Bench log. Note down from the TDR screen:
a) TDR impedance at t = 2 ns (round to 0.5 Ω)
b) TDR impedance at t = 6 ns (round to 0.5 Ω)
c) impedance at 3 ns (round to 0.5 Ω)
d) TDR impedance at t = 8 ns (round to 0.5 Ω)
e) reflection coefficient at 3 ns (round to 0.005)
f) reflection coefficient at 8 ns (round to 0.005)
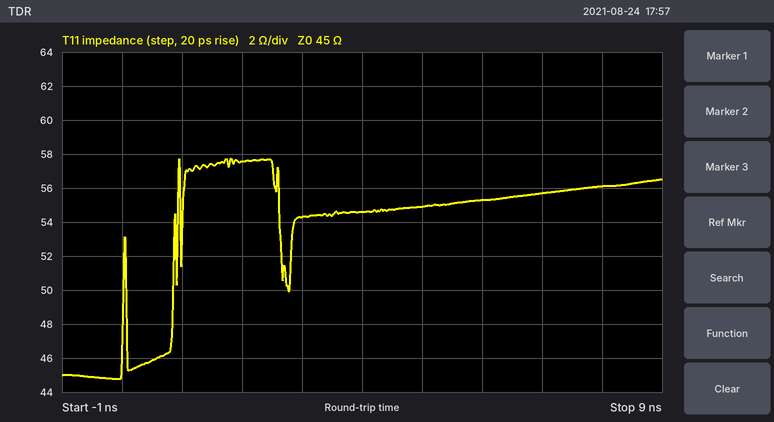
57.5 Ω
55.5 Ω
54.5 Ω
56.0 Ω
+0.095
+0.110
